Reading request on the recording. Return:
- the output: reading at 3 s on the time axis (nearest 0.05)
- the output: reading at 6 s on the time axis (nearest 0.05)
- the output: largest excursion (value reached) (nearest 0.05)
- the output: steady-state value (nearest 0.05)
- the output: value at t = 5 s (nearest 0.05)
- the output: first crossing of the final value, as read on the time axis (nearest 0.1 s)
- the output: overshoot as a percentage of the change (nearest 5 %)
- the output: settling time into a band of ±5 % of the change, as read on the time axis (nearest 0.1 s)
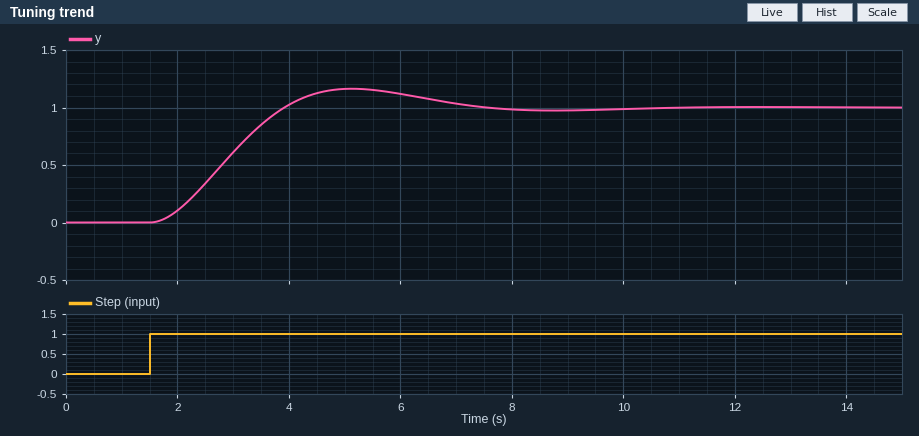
0.60
1.10
1.15
1.00
1.15
3.9 s
15 %
6.8 s
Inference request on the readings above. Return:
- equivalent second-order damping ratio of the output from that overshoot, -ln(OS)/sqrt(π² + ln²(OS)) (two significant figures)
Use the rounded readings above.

0.52
